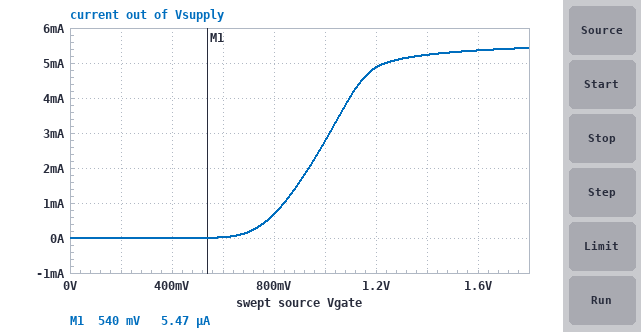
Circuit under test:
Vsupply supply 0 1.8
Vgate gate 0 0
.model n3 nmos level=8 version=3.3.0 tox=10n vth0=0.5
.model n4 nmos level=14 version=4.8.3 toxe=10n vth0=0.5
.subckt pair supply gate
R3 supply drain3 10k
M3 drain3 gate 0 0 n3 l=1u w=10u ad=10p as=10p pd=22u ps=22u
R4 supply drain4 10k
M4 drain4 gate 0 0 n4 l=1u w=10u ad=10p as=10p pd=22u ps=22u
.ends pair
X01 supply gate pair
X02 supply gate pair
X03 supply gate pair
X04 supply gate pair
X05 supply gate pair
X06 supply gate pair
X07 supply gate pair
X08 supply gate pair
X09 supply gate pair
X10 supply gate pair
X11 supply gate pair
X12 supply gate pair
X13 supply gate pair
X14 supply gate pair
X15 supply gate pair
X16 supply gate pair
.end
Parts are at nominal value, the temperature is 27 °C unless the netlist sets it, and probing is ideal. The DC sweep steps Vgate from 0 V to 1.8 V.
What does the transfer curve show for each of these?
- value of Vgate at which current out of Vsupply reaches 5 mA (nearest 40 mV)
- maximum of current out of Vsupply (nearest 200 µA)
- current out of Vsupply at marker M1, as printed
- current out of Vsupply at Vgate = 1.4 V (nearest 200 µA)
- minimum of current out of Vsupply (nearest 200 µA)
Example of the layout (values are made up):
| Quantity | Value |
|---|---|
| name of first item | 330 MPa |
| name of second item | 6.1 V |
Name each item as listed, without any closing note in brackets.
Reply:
| Quantity | Value |
|---|---|
| value of Vgate at which current out of Vsupply reaches 5 mA | 1.24 V |
| maximum of current out of Vsupply | 5.4 mA |
| current out of Vsupply at marker M1, as printed | 5.47 µA |
| current out of Vsupply at Vgate = 1.4 V | 5.2 mA |
| minimum of current out of Vsupply | 0 A |
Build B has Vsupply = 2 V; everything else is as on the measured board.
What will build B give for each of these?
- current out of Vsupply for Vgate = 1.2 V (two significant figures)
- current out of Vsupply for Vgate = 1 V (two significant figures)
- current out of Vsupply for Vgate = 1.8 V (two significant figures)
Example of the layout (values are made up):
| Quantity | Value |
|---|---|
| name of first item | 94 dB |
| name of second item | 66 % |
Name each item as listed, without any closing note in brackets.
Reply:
| Quantity | Value |
|---|---|
| current out of Vsupply for Vgate = 1.2 V | 5.2 mA |
| current out of Vsupply for Vgate = 1 V | 2.8 mA |
| current out of Vsupply for Vgate = 1.8 V | 6.0 mA |
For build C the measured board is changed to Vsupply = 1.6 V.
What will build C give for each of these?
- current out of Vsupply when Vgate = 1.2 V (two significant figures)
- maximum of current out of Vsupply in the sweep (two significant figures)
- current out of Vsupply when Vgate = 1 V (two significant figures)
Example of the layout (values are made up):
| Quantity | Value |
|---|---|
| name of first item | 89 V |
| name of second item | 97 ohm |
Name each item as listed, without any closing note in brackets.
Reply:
| Quantity | Value |
|---|---|
| current out of Vsupply when Vgate = 1.2 V | 4.4 mA |
| maximum of current out of Vsupply in the sweep | 4.8 mA |
| current out of Vsupply when Vgate = 1 V | 2.7 mA |
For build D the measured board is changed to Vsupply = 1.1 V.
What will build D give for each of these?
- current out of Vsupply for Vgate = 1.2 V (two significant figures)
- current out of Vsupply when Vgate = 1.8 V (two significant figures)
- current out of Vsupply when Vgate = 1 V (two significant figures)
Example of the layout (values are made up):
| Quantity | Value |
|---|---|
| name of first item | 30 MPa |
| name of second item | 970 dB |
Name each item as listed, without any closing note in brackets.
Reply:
| Quantity | Value |
|---|---|
| current out of Vsupply for Vgate = 1.2 V | 3.1 mA |
| current out of Vsupply when Vgate = 1.8 V | 3.3 mA |
| current out of Vsupply when Vgate = 1 V | 2.5 mA |
